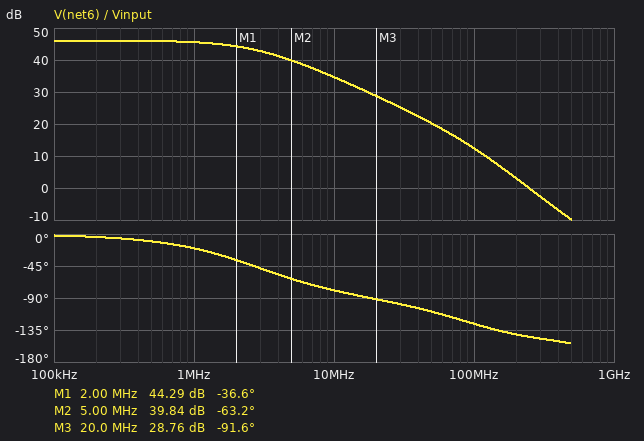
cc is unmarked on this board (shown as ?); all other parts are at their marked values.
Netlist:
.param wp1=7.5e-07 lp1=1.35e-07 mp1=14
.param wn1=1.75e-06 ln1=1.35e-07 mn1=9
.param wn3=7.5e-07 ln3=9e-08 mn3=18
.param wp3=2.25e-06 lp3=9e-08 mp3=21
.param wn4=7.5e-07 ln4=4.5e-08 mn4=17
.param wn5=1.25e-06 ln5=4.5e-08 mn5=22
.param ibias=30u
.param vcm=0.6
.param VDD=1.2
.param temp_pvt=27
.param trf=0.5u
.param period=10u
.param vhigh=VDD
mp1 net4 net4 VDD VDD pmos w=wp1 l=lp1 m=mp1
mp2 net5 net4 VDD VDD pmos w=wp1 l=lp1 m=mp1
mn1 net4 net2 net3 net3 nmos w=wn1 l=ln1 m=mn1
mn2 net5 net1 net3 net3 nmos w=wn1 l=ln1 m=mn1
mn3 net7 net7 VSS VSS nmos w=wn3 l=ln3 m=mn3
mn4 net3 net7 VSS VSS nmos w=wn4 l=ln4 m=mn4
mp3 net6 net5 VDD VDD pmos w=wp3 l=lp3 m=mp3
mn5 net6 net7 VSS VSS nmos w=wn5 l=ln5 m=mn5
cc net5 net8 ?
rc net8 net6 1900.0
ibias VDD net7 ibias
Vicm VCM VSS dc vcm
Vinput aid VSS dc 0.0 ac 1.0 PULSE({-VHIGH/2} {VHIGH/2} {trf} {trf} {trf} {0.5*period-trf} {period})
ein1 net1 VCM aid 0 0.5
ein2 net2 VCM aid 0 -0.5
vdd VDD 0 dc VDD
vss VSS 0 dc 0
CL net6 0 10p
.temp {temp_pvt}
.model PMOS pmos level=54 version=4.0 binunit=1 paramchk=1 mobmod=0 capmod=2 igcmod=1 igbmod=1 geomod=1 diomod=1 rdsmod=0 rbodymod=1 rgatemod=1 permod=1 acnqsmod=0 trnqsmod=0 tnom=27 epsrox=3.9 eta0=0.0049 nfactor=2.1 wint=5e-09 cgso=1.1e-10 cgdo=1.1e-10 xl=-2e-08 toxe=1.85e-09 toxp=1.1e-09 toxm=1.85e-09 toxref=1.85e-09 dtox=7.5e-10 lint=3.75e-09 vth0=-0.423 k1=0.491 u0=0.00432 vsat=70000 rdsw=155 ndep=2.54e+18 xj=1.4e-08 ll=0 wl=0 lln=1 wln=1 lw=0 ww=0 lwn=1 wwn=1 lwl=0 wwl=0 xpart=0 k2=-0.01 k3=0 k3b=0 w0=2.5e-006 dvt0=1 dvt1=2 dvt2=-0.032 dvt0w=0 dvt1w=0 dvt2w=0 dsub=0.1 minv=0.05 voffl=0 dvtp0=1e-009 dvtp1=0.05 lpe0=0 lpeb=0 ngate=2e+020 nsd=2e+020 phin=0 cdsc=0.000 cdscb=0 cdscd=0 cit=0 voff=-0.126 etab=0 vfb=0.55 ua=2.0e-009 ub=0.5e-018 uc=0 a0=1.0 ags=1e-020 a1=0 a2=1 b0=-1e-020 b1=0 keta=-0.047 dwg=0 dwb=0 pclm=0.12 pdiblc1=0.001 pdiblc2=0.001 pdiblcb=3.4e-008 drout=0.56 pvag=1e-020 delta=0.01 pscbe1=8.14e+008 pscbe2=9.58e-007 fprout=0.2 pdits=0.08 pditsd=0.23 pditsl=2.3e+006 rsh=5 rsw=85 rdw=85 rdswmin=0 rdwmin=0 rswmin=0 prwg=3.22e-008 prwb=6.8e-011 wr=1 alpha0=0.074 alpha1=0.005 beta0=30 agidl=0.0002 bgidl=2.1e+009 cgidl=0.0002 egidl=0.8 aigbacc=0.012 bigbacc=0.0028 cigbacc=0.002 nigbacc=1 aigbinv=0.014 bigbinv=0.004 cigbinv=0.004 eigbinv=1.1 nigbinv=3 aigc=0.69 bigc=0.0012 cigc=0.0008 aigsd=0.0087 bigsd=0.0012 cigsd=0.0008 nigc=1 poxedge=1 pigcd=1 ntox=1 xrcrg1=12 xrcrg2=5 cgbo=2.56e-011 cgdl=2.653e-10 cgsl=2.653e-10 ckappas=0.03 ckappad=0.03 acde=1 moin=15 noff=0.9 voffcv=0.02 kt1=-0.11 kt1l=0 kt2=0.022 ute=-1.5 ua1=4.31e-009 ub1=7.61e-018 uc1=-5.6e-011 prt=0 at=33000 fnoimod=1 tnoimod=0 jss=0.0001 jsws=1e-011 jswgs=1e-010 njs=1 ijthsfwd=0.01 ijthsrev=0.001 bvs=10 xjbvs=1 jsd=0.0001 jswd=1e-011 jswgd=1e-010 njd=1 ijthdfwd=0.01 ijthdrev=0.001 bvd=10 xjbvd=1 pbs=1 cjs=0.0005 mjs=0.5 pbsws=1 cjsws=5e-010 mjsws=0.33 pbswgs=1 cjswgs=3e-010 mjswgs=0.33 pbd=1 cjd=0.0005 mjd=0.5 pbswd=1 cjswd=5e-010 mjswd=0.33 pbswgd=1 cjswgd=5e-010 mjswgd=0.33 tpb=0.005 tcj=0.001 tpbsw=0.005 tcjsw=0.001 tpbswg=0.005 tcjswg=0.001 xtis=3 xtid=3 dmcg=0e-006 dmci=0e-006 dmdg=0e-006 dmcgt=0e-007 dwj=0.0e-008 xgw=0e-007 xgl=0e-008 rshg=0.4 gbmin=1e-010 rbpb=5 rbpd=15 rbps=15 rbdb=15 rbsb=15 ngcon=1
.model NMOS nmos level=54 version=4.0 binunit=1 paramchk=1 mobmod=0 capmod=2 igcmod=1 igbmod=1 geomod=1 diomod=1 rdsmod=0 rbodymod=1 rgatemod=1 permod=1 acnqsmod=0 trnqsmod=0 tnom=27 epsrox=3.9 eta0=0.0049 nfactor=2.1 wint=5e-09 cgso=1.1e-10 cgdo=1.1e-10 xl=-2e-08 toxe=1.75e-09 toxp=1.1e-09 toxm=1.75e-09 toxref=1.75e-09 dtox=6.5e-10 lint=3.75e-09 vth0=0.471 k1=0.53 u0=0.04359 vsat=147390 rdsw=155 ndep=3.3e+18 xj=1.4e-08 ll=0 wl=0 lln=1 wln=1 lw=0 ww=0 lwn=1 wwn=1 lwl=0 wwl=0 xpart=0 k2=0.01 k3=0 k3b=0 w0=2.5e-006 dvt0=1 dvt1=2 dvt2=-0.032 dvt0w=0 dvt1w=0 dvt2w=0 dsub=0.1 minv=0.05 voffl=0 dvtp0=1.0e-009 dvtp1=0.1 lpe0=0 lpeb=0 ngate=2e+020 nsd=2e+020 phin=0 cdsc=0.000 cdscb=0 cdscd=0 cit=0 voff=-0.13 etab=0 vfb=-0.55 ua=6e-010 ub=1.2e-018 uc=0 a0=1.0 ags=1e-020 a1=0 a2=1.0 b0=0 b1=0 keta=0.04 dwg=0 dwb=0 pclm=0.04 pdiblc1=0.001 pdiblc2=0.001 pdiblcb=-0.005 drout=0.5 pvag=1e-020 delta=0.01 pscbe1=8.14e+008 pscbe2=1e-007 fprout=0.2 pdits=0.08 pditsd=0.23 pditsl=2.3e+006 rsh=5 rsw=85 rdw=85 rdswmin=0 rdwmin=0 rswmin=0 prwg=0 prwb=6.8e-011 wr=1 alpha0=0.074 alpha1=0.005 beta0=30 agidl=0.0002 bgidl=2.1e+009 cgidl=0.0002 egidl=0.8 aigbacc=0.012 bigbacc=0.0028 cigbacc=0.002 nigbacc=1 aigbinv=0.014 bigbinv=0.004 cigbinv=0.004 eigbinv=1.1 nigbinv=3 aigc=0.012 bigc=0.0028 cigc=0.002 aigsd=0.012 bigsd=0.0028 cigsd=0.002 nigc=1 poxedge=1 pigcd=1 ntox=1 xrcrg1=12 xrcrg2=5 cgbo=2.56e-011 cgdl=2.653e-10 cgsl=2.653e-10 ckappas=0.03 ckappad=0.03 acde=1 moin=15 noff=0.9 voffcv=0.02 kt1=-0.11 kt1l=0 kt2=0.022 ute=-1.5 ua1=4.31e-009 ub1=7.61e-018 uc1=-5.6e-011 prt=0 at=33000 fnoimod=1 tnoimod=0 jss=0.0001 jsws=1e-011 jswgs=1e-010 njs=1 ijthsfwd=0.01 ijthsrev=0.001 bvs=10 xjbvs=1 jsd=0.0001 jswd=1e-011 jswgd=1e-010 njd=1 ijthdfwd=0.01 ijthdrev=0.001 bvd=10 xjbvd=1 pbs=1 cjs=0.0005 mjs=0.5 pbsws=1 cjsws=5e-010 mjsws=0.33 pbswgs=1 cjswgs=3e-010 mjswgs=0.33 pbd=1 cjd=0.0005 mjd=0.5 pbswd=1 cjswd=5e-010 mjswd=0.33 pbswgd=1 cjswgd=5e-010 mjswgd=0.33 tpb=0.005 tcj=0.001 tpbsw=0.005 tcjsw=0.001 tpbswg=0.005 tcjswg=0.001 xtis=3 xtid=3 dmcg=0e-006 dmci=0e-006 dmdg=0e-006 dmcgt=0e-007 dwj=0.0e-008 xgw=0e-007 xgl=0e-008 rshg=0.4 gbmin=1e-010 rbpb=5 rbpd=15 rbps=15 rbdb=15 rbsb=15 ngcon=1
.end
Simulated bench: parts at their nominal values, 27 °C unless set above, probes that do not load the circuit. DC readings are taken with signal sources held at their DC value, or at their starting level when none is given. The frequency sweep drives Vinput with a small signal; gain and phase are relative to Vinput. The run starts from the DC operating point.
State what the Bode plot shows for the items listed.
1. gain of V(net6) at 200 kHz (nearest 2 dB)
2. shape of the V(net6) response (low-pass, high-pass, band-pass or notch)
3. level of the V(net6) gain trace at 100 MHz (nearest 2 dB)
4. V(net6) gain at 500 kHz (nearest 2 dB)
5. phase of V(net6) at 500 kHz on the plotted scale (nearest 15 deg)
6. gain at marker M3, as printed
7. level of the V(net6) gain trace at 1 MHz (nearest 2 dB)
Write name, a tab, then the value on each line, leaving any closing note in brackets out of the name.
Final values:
gain of V(net6) at 200 kHz	46 dB
shape of the V(net6) response	low-pass
level of the V(net6) gain trace at 100 MHz	12 dB
V(net6) gain at 500 kHz	46 dB
phase of V(net6) at 500 kHz on the plotted scale	-15 deg
gain at marker M3, as printed	28.76 dB
level of the V(net6) gain trace at 1 MHz	46 dB
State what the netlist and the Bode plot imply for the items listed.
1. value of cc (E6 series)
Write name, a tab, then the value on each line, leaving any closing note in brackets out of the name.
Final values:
value of cc	220 fF
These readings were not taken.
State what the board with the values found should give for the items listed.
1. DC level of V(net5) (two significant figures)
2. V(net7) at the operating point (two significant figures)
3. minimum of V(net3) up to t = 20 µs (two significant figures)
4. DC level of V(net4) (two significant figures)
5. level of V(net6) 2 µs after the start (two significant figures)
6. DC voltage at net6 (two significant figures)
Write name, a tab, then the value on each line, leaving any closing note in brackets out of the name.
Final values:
DC level of V(net5)	600 mV
V(net7) at the operating point	370 mV
minimum of V(net3) up to t = 20 µs	3.2 mV
DC level of V(net4)	600 mV
level of V(net6) 2 µs after the start	1.0 V
DC voltage at net6	380 mV
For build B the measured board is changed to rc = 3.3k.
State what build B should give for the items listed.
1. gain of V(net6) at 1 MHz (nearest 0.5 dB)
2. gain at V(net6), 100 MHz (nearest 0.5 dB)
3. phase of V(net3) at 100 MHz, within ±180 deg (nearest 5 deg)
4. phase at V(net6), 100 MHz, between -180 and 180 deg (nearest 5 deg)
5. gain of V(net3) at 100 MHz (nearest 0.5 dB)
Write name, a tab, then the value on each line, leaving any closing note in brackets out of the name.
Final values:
gain of V(net6) at 1 MHz	45.5 dB
gain at V(net6), 100 MHz	13.0 dB
phase of V(net3) at 100 MHz, within ±180 deg	145 deg
phase at V(net6), 100 MHz, between -180 and 180 deg	-120 deg
gain of V(net3) at 100 MHz	-25.0 dB
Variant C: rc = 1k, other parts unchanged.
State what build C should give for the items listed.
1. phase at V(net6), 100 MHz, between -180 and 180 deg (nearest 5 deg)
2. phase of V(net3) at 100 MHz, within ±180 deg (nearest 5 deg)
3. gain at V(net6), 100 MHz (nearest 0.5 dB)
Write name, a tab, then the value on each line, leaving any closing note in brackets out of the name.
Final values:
phase at V(net6), 100 MHz, between -180 and 180 deg	-130 deg
phase of V(net3) at 100 MHz, within ±180 deg	135 deg
gain at V(net6), 100 MHz	12.0 dB
